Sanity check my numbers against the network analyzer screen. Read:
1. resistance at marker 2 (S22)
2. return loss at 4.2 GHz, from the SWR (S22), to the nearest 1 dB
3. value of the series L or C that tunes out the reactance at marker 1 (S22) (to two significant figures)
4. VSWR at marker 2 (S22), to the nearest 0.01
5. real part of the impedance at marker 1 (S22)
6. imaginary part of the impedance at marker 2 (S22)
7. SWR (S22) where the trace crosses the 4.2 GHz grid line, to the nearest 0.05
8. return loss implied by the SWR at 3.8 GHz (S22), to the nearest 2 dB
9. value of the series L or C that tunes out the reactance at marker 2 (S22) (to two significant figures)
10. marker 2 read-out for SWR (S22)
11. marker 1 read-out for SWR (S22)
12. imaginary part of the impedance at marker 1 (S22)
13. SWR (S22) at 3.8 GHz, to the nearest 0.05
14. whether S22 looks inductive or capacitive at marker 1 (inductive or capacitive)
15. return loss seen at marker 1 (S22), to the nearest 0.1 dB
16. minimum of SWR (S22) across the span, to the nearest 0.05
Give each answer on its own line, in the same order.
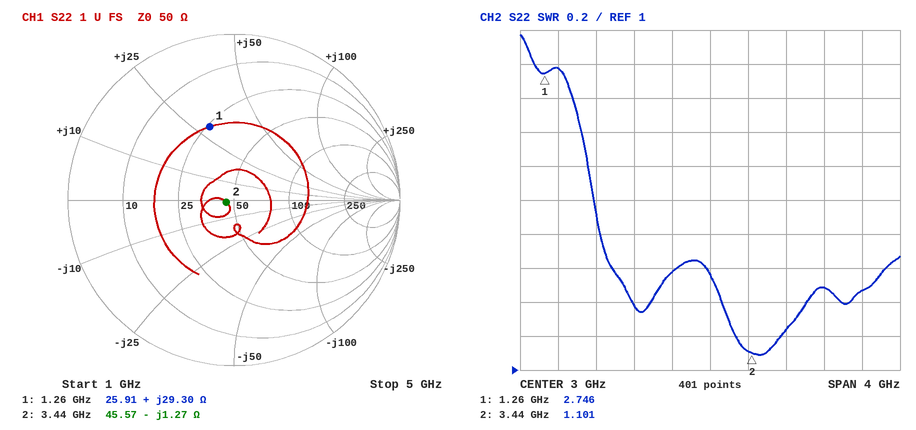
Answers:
45.57 Ω
14 dB
4.3 pF
1.10
25.91 Ω
-1.27 Ω
1.50
20 dB
59 pH
1.101
2.746
+29.30 Ω
1.25
inductive
6.6 dB
1.10
